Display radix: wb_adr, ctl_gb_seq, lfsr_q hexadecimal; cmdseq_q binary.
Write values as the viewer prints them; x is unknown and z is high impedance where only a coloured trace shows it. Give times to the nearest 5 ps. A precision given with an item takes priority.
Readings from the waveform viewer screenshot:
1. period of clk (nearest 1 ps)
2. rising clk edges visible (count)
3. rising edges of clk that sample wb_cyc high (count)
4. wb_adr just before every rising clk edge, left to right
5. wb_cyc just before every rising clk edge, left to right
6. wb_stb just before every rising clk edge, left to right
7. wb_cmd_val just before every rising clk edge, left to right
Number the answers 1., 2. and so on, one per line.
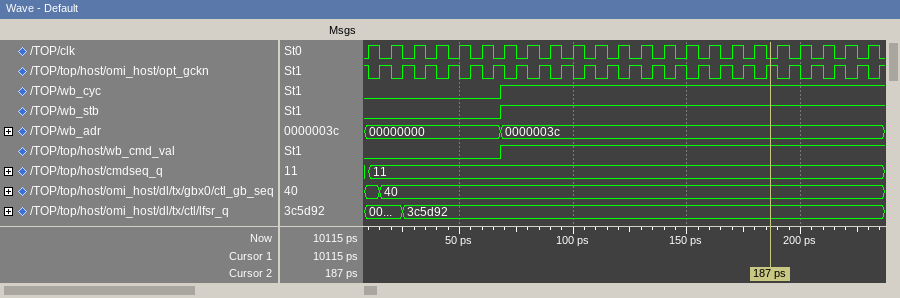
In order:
1. 10 ps
2. 23
3. 17
4. 00000000, 00000000, 00000000, 00000000, 00000000, 00000000, 0000003c, 0000003c, 0000003c, 0000003c, 0000003c, 0000003c, 0000003c, 0000003c, 0000003c, 0000003c, 0000003c, 0000003c, 0000003c, 0000003c, 0000003c, 0000003c, 0000003c
5. 0 0 0 0 0 0 1 1 1 1 1 1 1 1 1 1 1 1 1 1 1 1 1
6. 0 0 0 0 0 0 1 1 1 1 1 1 1 1 1 1 1 1 1 1 1 1 1
7. 0 0 0 0 0 0 1 1 1 1 1 1 1 1 1 1 1 1 1 1 1 1 1
